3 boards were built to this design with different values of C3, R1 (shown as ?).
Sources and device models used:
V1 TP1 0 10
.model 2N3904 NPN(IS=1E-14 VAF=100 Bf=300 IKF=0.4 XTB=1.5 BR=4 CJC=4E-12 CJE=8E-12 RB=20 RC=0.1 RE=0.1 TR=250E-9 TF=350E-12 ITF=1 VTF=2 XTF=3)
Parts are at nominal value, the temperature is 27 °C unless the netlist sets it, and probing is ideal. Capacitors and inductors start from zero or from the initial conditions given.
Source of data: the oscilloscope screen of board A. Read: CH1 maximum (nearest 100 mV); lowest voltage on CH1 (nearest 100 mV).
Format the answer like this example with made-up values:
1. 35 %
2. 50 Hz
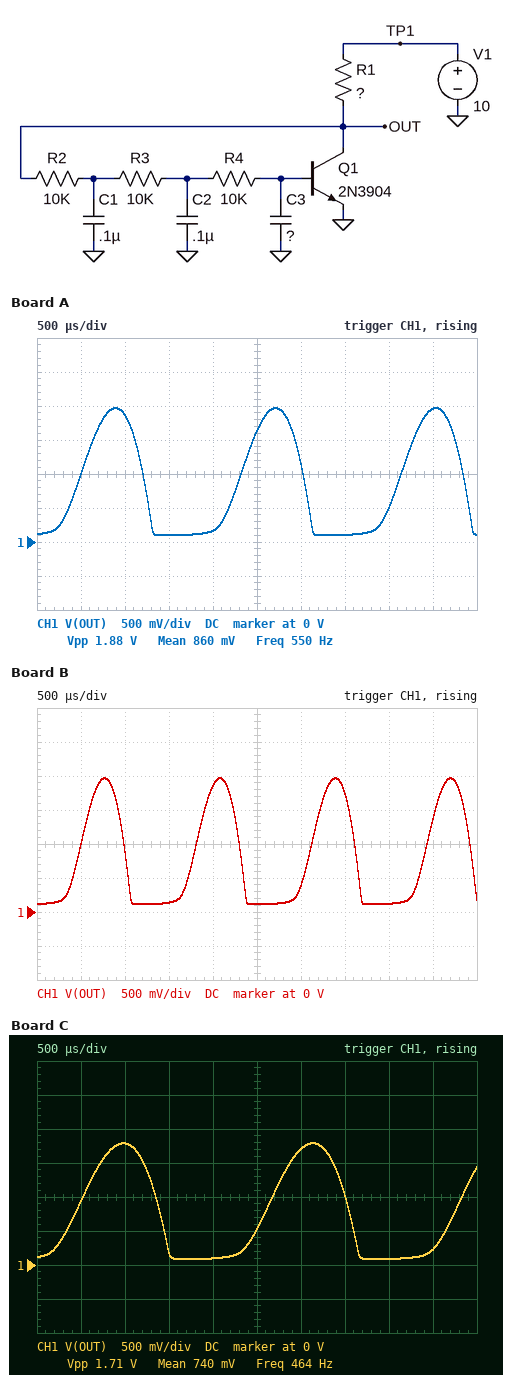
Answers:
1. 2.0 V
2. 100 mV
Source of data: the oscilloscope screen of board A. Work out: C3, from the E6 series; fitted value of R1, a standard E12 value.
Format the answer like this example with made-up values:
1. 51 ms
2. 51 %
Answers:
1. 150 nF
2. 10 kΩ
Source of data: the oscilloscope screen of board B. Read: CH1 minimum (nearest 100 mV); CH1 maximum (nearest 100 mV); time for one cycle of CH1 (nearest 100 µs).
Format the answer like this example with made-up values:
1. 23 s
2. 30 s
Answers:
1. 100 mV
2. 2.0 V
3. 1.3 ms
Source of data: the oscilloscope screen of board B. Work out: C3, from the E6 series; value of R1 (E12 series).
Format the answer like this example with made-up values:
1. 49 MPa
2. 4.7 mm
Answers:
1. 47 nF
2. 10 kΩ
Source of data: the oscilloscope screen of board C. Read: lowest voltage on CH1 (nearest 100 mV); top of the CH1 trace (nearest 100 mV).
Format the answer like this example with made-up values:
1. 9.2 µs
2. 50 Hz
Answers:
1. 100 mV
2. 1.8 V
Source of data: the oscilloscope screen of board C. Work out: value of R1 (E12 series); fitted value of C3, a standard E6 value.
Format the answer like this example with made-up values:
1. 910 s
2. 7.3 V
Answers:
1. 15 kΩ
2. 220 nF
